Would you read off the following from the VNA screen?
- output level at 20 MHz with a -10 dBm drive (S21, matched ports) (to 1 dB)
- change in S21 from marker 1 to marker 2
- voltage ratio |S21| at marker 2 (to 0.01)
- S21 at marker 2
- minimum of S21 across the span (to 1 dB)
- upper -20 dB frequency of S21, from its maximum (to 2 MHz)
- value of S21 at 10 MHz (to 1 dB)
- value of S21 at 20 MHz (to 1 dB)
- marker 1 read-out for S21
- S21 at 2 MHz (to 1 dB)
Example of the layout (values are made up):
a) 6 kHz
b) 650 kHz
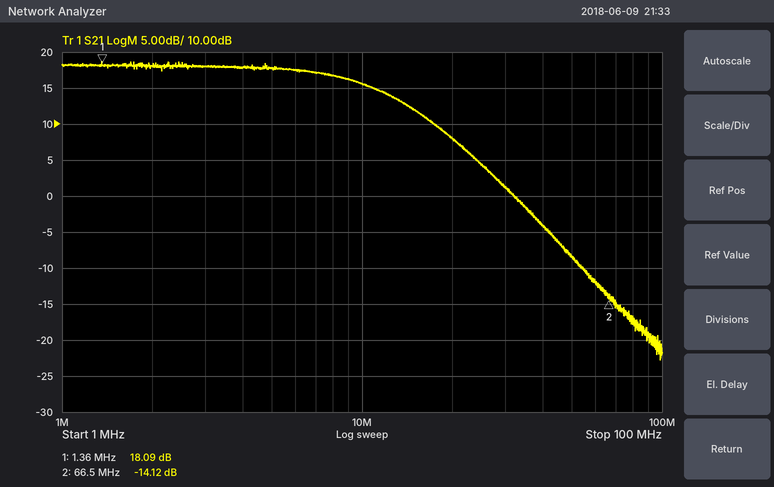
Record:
a) -2 dBm
b) -32.21 dB
c) 0.20
d) -14.12 dB
e) -23 dB
f) 34 MHz
g) 16 dB
h) 8 dB
i) 18.09 dB
j) 18 dB
